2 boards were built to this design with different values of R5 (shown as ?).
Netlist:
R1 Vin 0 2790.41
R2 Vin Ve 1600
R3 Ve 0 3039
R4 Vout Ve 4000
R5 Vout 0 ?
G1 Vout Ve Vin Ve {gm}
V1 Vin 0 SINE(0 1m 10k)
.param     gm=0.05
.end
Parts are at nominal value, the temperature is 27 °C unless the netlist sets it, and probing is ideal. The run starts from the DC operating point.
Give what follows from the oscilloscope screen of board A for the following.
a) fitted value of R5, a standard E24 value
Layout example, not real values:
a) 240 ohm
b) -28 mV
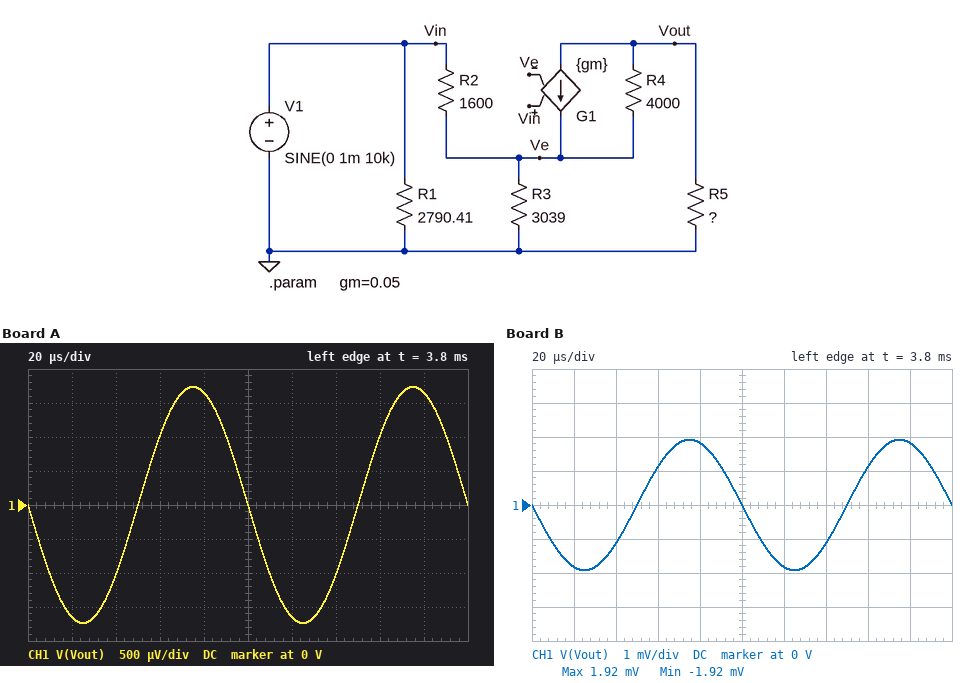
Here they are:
a) 5.6 kΩ
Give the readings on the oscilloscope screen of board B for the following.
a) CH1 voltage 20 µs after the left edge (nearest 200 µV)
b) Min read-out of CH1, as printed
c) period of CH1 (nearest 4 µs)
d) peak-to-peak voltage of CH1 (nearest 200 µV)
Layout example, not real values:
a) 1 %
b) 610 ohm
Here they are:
a) -1.8 mV
b) -1.92 mV
c) 100 µs
d) 3.8 mV
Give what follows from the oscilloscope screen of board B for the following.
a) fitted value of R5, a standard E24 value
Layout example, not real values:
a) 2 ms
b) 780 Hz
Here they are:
a) 6.2 kΩ
